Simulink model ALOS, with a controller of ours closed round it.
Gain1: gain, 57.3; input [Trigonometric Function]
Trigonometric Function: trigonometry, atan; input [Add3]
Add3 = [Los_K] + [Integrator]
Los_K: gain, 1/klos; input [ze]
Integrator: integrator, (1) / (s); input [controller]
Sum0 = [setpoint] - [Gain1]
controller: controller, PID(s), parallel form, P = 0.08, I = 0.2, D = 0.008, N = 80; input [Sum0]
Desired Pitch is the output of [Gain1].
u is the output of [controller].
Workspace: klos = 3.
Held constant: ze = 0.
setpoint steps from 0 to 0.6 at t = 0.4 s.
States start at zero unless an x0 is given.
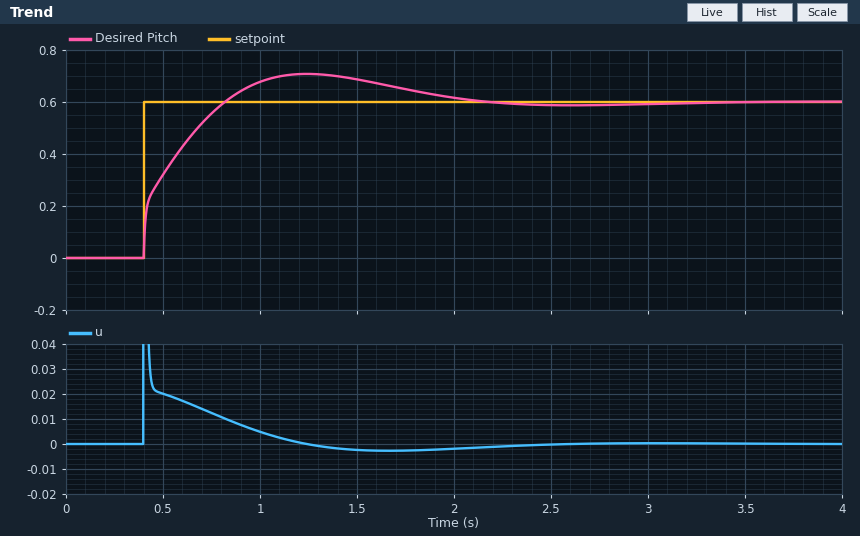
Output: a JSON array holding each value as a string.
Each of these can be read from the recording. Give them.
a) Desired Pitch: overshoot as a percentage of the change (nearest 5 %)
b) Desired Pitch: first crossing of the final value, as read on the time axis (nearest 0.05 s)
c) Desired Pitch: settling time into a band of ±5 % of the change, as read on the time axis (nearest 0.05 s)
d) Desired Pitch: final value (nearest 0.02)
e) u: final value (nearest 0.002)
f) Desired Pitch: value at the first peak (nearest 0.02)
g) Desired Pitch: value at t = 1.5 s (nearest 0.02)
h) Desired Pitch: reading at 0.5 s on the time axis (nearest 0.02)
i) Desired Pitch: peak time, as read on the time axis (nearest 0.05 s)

["20 %", "0.80 s", "1.90 s", "0.60", "0.000", "0.70", "0.68", "0.32", "1.25 s"]
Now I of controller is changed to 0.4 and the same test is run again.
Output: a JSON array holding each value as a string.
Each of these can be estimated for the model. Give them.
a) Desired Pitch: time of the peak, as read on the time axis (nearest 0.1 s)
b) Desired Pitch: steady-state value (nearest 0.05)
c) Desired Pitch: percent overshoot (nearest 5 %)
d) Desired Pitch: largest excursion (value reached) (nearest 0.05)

["1.0 s", "0.60", "25 %", "0.75"]
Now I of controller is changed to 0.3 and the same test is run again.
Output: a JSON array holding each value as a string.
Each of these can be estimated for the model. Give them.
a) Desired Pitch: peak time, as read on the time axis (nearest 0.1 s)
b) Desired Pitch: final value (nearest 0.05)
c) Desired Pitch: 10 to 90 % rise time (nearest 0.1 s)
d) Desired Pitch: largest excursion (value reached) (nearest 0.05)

["1.1 s", "0.60", "0.3 s", "0.75"]
